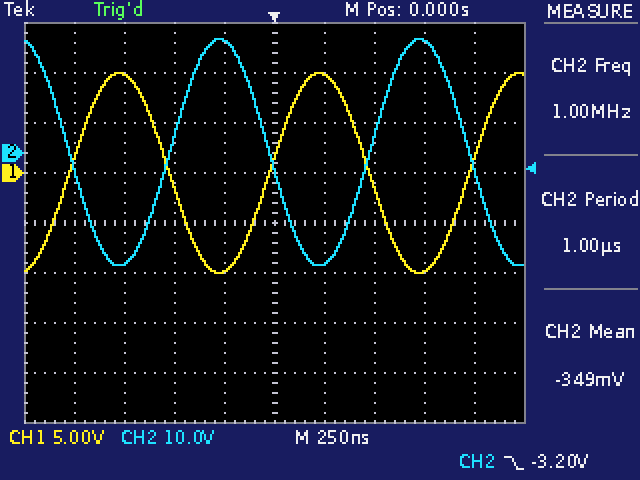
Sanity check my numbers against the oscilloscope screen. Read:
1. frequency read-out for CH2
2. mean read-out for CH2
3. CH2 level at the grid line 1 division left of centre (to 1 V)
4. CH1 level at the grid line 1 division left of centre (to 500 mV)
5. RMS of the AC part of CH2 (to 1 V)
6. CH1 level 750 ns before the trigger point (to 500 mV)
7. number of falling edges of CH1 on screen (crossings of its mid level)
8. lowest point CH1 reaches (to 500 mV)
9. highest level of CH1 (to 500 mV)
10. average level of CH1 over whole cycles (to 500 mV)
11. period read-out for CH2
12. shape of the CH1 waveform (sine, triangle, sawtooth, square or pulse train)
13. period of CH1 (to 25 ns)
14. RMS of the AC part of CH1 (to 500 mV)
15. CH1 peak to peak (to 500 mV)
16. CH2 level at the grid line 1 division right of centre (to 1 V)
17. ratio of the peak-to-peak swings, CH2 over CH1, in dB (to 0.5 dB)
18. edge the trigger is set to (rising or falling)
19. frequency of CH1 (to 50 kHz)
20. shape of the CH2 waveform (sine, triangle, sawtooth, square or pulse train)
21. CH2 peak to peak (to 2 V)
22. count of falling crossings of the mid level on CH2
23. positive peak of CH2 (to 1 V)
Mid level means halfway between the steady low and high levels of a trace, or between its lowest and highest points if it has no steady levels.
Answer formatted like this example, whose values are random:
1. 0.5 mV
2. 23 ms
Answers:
1. 1.00 MHz
2. -349 mV
3. 22 V
4. -10.0 V
5. 16 V
6. 10.0 V
7. 2
8. -10.0 V
9. 10.0 V
10. 0.0 V
11. 1.00 µs
12. sine
13. 1.000 µs
14. 7.0 V
15. 20.0 V
16. -22 V
17. 7.0 dB
18. falling
19. 1.00 MHz
20. sine
21. 46 V
22. 3
23. 23 V
